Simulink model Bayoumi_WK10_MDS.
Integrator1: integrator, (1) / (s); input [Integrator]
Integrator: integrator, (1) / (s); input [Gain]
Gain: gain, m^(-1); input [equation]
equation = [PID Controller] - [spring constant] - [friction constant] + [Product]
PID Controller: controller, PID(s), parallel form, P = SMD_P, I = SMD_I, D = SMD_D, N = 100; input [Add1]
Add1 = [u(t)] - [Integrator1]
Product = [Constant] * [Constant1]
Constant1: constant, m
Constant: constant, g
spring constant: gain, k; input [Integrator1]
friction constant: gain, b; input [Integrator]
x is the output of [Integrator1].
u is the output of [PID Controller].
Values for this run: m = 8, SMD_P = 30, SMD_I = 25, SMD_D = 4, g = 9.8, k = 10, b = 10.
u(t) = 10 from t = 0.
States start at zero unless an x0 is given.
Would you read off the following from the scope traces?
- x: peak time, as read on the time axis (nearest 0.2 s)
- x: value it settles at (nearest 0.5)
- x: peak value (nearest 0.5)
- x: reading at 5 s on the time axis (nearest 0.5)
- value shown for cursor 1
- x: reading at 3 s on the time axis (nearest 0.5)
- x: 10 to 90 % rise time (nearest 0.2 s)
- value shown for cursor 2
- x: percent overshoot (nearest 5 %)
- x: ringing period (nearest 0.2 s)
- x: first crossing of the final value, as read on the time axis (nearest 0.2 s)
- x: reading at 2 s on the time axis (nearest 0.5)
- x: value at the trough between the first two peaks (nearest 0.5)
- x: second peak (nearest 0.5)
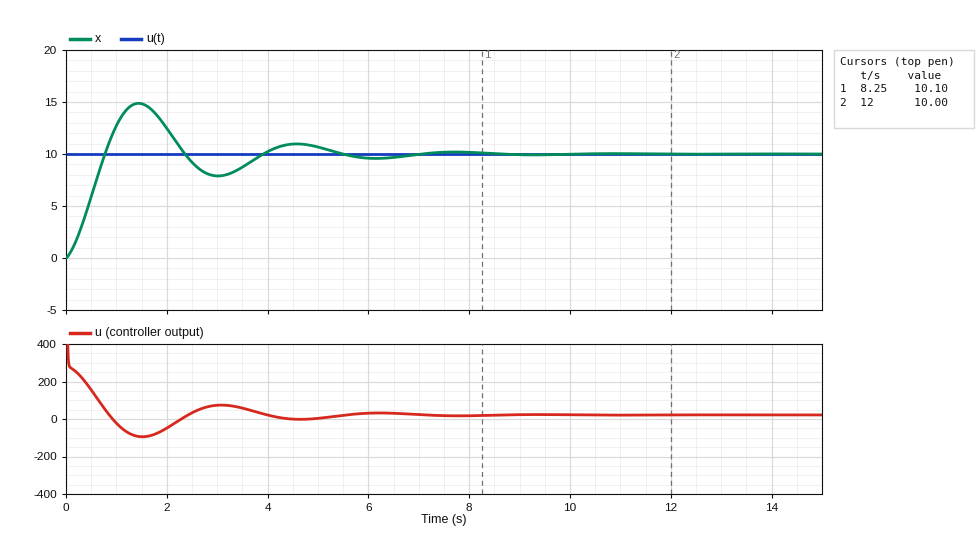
1.4 s
10.0
15.0
10.5
10.10
8.0
0.6 s
10.00
50 %
3.2 s
0.8 s
12.5
8.0
11.0
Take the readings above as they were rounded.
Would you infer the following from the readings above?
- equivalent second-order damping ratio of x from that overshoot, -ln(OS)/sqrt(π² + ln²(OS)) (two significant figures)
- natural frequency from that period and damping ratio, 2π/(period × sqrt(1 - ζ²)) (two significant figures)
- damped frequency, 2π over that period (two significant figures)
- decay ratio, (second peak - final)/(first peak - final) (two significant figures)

0.22
2.0 rad/s
2.0 rad/s
0.20
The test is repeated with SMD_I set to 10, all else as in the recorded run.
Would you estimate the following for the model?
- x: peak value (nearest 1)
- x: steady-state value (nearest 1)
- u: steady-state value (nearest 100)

13
10
0
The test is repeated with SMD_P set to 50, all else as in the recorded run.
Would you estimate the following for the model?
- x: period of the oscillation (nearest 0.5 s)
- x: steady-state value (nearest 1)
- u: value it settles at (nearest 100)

2.5 s
10
0
